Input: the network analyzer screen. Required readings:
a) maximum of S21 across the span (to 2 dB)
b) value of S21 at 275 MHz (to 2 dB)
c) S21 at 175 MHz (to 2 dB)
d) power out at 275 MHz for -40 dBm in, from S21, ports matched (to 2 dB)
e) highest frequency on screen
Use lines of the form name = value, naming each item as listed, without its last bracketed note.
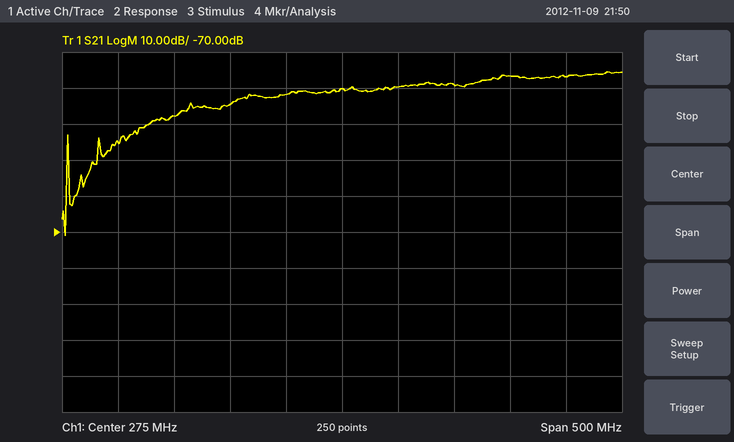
maximum of S21 across the span = -26 dB
value of S21 at 275 MHz = -30 dB
S21 at 175 MHz = -34 dB
power out at 275 MHz for -40 dBm in, from S21, ports matched = -70 dBm
highest frequency on screen = 525 MHz
